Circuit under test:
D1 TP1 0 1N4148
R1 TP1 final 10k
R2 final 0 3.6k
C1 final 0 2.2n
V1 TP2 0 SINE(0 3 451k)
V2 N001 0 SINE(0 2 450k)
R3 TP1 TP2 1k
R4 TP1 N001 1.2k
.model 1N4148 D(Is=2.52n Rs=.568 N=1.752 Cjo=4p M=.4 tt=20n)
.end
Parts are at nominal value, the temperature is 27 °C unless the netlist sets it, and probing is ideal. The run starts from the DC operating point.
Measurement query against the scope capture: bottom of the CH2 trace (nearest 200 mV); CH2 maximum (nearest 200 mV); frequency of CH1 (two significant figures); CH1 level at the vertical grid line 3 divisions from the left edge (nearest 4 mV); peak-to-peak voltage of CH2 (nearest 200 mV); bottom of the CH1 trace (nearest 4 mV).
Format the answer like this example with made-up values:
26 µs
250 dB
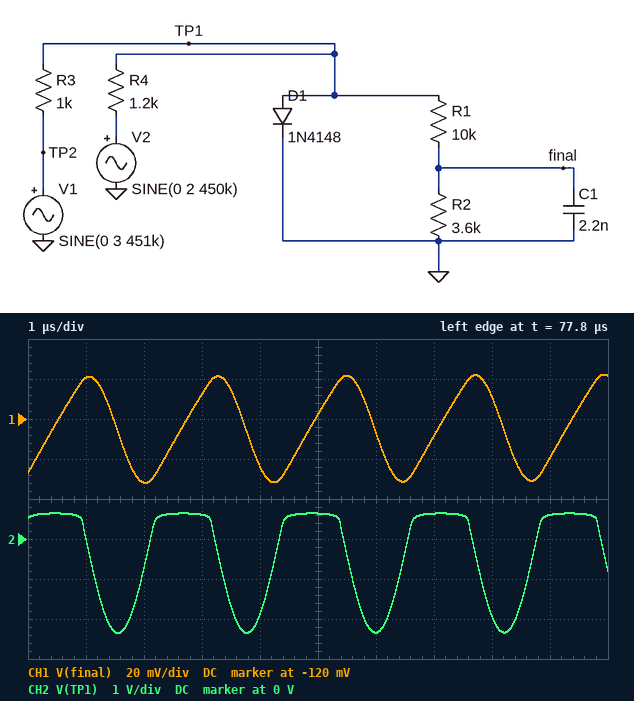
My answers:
-2.4 V
600 mV
450 kHz
-108 mV
3.0 V
-152 mV
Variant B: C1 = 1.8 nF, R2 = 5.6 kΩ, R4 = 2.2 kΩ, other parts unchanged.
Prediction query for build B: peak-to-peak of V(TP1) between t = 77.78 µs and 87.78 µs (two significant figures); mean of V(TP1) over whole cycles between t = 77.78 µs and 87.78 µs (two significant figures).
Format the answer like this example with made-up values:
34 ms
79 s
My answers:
3.1 V
-510 mV
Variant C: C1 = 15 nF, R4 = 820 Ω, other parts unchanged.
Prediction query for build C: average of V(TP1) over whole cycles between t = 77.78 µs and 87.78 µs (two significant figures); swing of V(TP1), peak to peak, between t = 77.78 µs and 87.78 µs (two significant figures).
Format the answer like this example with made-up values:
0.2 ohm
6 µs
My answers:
-440 mV
2.9 V
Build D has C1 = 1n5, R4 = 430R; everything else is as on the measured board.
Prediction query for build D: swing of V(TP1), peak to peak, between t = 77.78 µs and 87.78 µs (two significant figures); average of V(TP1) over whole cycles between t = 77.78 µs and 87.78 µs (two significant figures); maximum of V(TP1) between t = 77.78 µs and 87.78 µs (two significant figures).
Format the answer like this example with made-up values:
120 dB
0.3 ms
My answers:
2.8 V
-400 mV
660 mV
